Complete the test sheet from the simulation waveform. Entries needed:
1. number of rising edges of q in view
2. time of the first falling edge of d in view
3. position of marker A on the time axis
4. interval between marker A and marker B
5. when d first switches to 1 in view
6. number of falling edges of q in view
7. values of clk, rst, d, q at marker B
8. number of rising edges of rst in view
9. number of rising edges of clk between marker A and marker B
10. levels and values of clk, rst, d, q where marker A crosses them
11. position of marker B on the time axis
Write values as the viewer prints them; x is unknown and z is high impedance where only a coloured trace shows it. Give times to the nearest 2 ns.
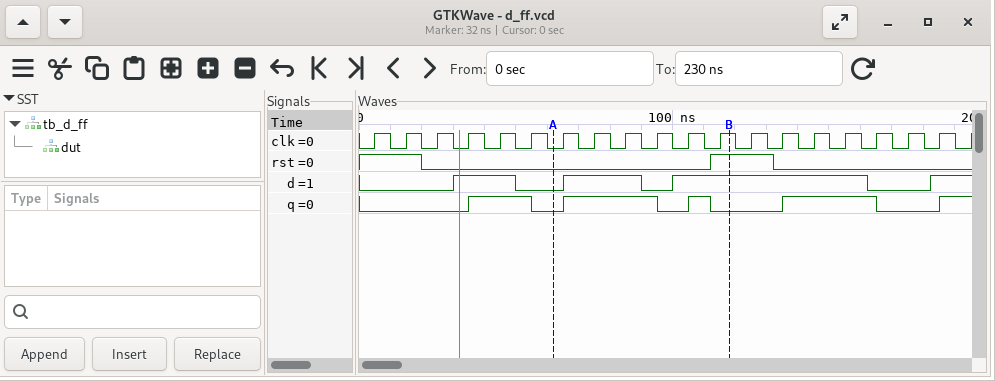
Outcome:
5
50 ns
62 ns
56 ns
30 ns
4
clk=1, rst=1, d=1, q=0
1
6
clk=0, rst=0, d=0, q=0
118 ns
